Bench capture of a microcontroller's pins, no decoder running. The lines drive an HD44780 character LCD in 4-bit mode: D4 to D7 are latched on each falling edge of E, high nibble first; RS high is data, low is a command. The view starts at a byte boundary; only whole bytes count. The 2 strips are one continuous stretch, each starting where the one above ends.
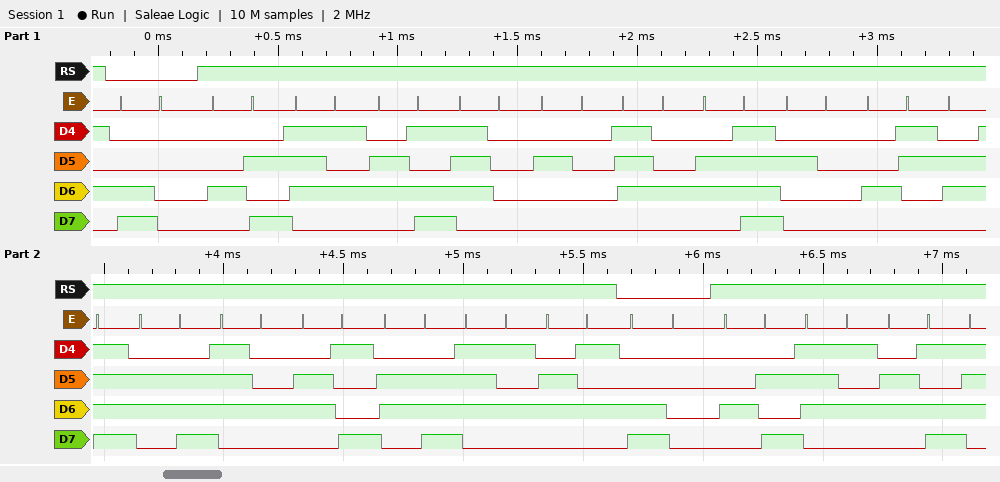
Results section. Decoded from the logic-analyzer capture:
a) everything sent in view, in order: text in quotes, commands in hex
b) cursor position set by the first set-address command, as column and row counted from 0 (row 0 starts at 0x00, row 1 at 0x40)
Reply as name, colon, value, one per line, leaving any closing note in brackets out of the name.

everything sent in view, in order: text in quotes, commands in hex: 0xC0 "Jump to Continue" 0xC0 "Jum"
cursor position set by the first set-address command, as column and row counted from 0: column 0, row 1
